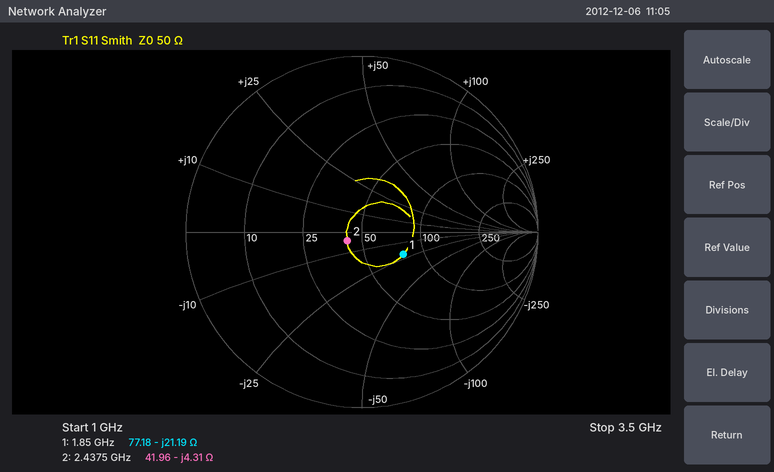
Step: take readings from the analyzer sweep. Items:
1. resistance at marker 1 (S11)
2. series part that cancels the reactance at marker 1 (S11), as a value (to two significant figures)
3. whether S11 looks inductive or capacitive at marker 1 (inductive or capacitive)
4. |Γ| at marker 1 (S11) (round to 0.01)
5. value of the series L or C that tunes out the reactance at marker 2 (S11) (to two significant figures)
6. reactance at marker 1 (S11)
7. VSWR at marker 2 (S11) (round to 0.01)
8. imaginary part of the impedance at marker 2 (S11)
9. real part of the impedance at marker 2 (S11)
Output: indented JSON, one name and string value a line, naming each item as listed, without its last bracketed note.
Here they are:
{
  "resistance at marker 1": "77.18 Ω",
  "series part that cancels the reactance at marker 1 (S11), as a value": "1.8 nH",
  "whether S11 looks inductive or capacitive at marker 1": "capacitive",
  "|Γ| at marker 1 (S11)": "0.27",
  "value of the series L or C that tunes out the reactance at marker 2 (S11)": "280 pH",
  "reactance at marker 1": "-21.19 Ω",
  "VSWR at marker 2 (S11)": "1.22",
  "imaginary part of the impedance at marker 2": "-4.31 Ω",
  "real part of the impedance at marker 2": "41.96 Ω"
}
